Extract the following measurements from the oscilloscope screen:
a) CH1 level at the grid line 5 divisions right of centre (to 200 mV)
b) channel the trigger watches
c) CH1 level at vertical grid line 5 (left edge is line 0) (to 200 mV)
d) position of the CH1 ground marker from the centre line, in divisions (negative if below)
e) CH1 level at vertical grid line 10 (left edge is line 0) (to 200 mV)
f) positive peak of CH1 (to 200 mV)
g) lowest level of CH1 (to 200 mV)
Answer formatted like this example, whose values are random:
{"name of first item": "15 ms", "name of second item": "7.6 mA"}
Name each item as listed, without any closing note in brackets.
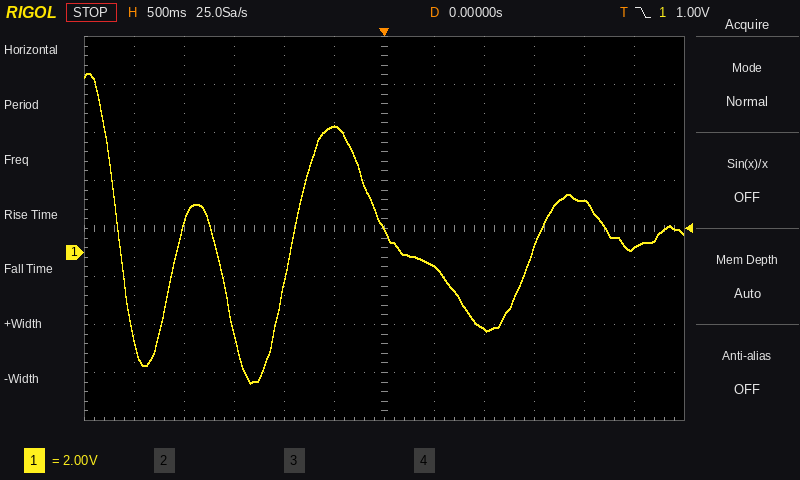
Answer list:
{"CH1 level at the grid line 5 divisions right of centre": "200 mV", "channel the trigger watches": "CH1", "CH1 level at vertical grid line 5 (left edge is line 0)": "5.2 V", "position of the CH1 ground marker from the centre line, in divisions": "-0.5 div", "CH1 level at vertical grid line 10 (left edge is line 0)": "2.2 V", "positive peak of CH1": "7.4 V", "lowest level of CH1": "-5.4 V"}
